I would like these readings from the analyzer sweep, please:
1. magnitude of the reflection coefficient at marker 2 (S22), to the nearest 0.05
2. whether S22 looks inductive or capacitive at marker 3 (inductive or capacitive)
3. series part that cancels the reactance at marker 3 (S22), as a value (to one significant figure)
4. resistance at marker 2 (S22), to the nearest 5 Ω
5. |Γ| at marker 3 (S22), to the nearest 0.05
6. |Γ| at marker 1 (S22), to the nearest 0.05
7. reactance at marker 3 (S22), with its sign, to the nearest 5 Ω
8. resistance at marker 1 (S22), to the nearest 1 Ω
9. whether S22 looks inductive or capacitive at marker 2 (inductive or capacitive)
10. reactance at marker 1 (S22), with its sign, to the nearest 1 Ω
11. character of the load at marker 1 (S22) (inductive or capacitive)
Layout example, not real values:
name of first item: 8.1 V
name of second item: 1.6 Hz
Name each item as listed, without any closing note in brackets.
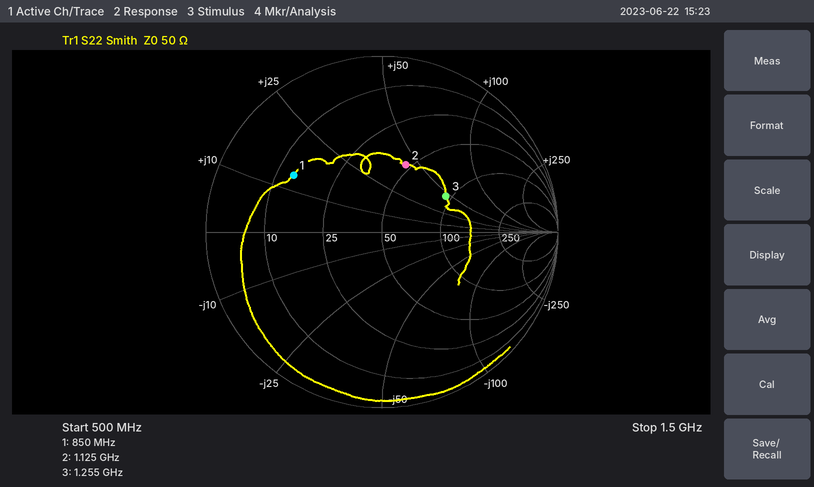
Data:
magnitude of the reflection coefficient at marker 2 (S22), to the nearest 0.05: 0.40
whether S22 looks inductive or capacitive at marker 3: inductive
series part that cancels the reactance at marker 3 (S22), as a value: 3 pF
resistance at marker 2 (S22), to the nearest 5 Ω: 45 Ω
|Γ| at marker 3 (S22), to the nearest 0.05: 0.40
|Γ| at marker 1 (S22), to the nearest 0.05: 0.60
reactance at marker 3 (S22), with its sign, to the nearest 5 Ω: +45 Ω
resistance at marker 1 (S22), to the nearest 1 Ω: 14 Ω
whether S22 looks inductive or capacitive at marker 2: inductive
reactance at marker 1 (S22), with its sign, to the nearest 1 Ω: +14 Ω
character of the load at marker 1 (S22): inductive
